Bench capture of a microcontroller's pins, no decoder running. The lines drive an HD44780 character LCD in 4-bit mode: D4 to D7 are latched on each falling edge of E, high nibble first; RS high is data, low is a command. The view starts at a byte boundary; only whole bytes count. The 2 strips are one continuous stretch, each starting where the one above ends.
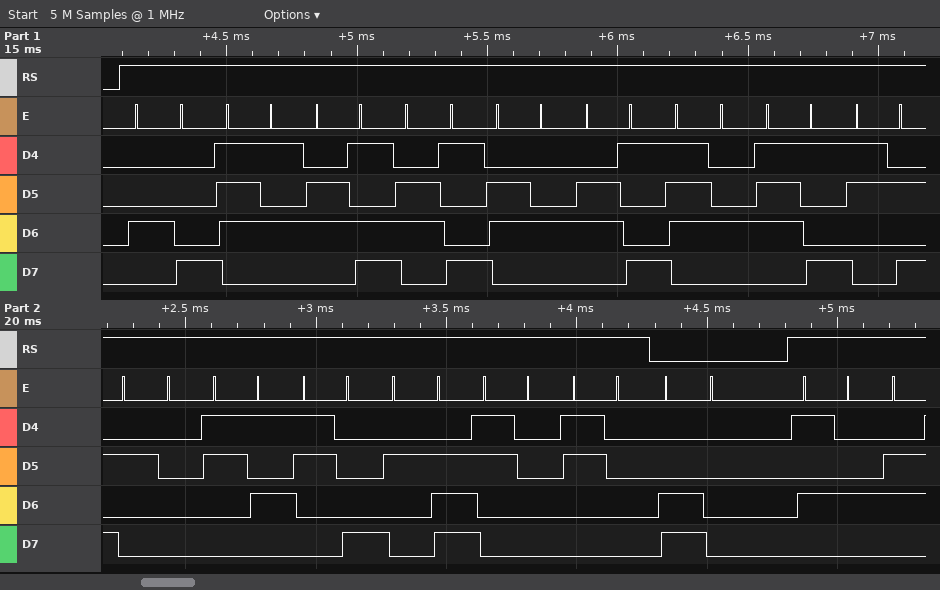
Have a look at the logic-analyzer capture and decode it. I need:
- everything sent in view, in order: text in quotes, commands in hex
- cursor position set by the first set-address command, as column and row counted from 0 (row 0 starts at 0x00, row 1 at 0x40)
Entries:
"Humidity: 58.00" 0xC0 "T"
column 0, row 1
